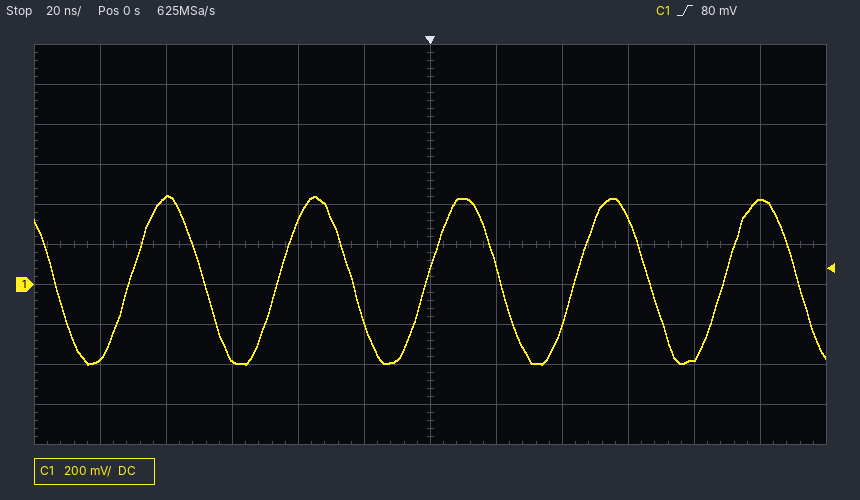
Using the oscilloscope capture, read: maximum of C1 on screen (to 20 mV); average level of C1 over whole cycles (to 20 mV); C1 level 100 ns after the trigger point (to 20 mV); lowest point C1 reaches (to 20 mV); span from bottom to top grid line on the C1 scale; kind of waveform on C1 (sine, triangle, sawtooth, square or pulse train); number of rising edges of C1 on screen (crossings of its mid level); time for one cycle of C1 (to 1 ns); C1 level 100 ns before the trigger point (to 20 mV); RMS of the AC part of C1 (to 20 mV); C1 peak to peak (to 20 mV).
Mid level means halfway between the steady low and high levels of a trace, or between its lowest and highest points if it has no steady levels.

440 mV
20 mV
420 mV
-400 mV
2 V
sine
5
45 ns
-380 mV
300 mV
840 mV
